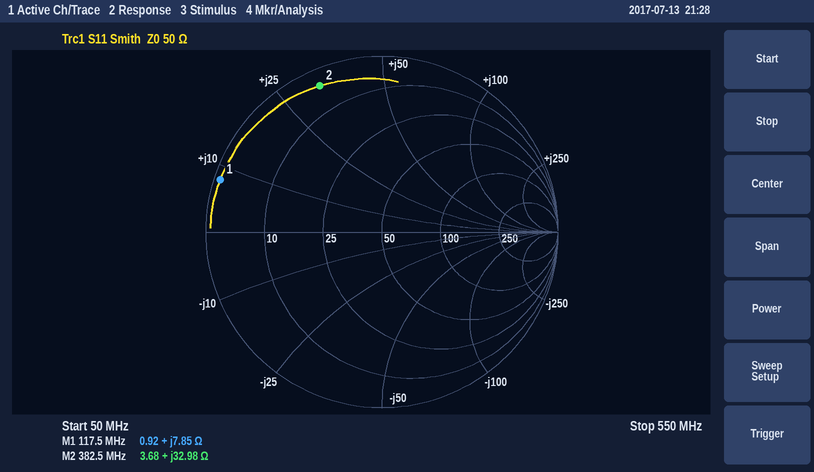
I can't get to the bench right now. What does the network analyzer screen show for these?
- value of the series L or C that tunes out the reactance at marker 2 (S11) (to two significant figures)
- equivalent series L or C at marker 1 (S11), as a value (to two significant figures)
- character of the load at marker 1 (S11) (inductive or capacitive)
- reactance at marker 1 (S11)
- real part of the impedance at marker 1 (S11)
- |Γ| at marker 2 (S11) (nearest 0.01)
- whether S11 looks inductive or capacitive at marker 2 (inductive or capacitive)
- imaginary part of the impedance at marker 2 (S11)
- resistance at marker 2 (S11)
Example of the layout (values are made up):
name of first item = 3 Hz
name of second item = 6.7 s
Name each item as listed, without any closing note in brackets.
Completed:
value of the series L or C that tunes out the reactance at marker 2 (S11) = 13 pF
equivalent series L or C at marker 1 (S11), as a value = 11 nH
character of the load at marker 1 (S11) = inductive
reactance at marker 1 = +7.85 Ω
real part of the impedance at marker 1 = 0.92 Ω
|Γ| at marker 2 (S11) = 0.90
whether S11 looks inductive or capacitive at marker 2 = inductive
imaginary part of the impedance at marker 2 = +32.98 Ω
resistance at marker 2 = 3.68 Ω
